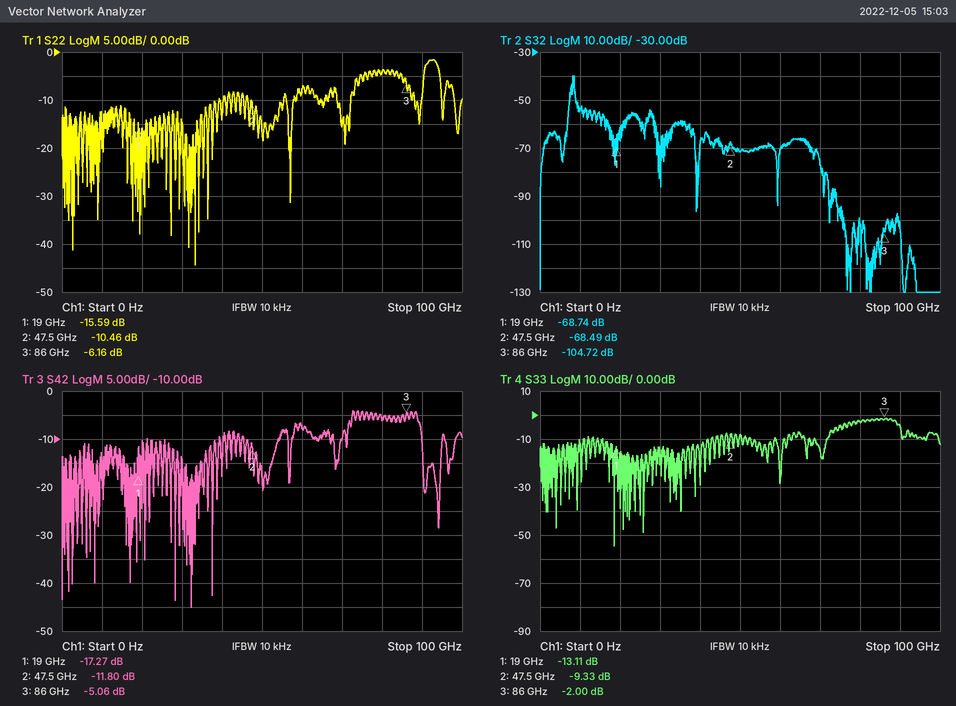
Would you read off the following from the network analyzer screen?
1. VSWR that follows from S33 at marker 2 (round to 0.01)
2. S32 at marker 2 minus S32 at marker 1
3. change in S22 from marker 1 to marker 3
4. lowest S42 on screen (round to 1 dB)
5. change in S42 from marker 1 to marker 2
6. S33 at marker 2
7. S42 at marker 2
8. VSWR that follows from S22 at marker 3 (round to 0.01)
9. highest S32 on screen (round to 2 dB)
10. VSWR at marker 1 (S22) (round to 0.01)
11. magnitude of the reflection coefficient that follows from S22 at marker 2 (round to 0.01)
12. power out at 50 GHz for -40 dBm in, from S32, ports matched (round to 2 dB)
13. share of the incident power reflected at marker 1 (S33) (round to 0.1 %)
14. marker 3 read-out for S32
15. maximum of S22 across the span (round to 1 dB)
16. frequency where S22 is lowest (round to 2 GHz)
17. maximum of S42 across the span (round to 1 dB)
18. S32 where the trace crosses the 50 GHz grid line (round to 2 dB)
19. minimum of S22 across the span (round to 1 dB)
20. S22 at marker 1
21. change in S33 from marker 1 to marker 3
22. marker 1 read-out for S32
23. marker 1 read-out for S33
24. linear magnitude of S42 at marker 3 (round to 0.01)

2.04
0.25 dB
9.43 dB
-45 dB
5.47 dB
-9.33 dB
-11.80 dB
2.94
-40 dB
1.40
0.30
-112 dBm
4.9 %
-104.72 dB
-2 dB
34 GHz
-4 dB
-72 dB
-44 dB
-15.59 dB
11.11 dB
-68.74 dB
-13.11 dB
0.56
